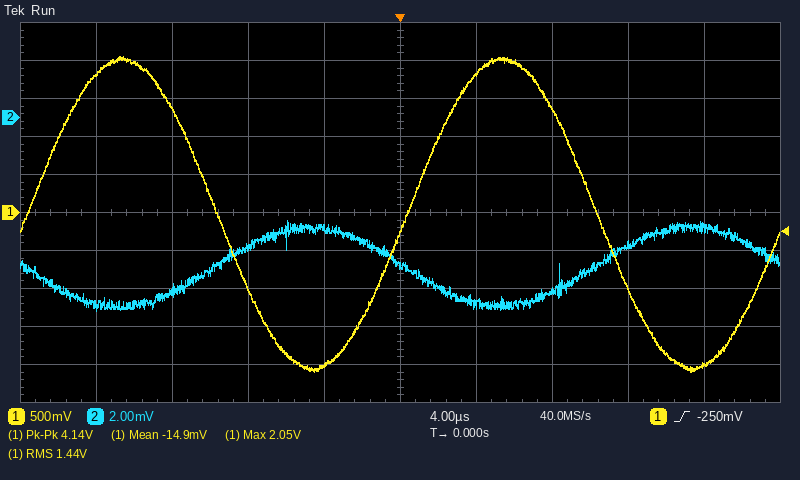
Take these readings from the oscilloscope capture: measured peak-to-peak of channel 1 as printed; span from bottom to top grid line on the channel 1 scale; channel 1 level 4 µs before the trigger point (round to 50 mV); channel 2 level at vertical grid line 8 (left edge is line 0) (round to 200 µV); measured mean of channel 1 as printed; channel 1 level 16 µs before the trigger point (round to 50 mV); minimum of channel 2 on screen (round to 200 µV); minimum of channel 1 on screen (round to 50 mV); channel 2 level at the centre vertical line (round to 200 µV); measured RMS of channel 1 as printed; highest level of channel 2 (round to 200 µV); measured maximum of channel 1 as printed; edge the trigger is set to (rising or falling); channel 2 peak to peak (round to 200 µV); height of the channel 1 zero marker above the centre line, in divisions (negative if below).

4.14 V
5 V
-2.00 V
-6.6 mV
-14.9 mV
1.80 V
-10.2 mV
-2.10 V
-7.8 mV
1.44 V
-5.4 mV
2.05 V
rising
4.8 mV
0.0 div
